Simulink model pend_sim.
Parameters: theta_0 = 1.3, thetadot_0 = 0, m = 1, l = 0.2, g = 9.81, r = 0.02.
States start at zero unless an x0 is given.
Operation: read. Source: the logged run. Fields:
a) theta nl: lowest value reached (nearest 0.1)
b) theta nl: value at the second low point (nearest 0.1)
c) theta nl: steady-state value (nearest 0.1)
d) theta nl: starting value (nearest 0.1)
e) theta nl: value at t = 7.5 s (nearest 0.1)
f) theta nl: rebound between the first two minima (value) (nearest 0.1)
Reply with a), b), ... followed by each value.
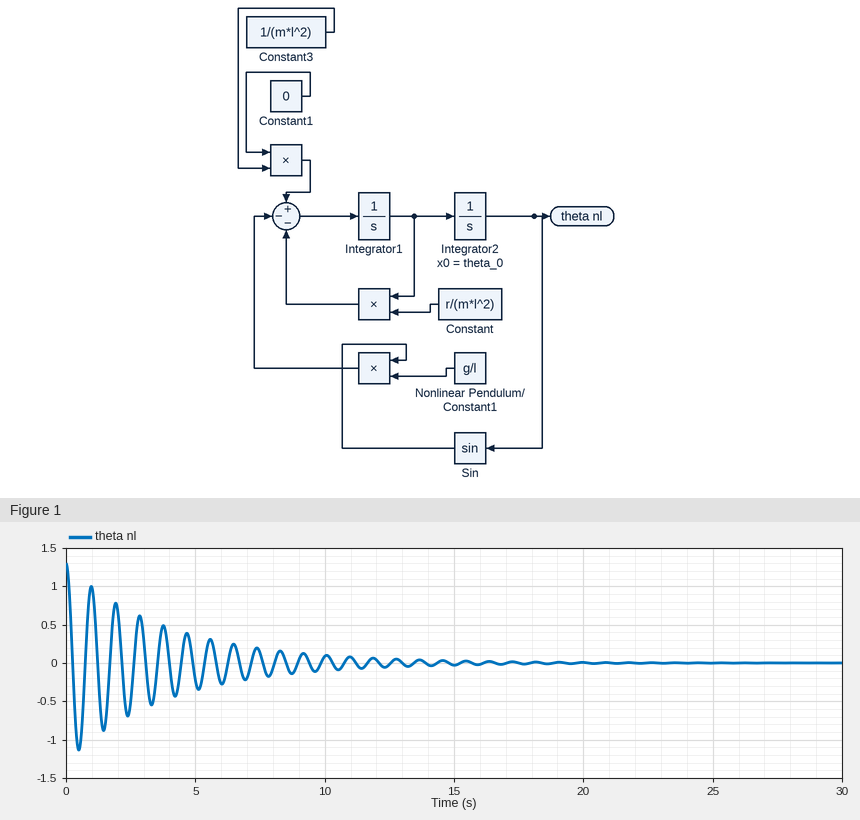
a) -1.1
b) -0.9
c) 0.0
d) 1.3
e) 0.1
f) 1.0
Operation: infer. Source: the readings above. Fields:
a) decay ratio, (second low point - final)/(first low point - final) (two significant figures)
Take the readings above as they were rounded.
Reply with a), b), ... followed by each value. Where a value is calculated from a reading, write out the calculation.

a) (-0.9 - 0) / (-1.1 - 0) = 0.82
